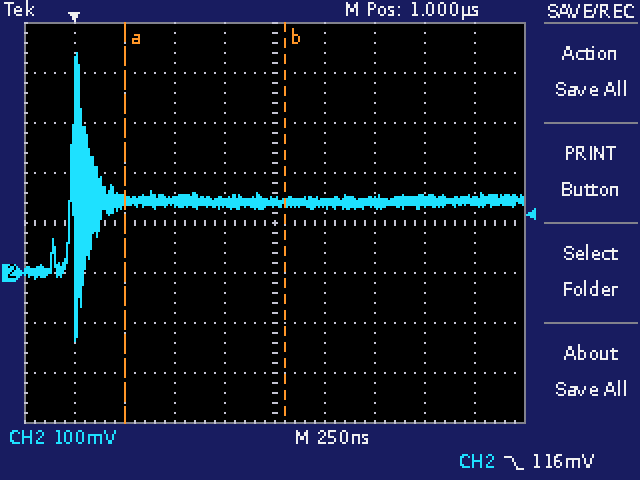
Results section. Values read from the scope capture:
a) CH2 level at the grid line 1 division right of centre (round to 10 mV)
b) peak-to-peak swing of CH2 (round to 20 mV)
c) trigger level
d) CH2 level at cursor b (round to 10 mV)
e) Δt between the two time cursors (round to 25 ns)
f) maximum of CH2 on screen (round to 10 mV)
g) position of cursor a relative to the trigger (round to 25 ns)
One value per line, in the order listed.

140 mV
580 mV
116 mV
140 mV
800 ns
440 mV
+250 ns
